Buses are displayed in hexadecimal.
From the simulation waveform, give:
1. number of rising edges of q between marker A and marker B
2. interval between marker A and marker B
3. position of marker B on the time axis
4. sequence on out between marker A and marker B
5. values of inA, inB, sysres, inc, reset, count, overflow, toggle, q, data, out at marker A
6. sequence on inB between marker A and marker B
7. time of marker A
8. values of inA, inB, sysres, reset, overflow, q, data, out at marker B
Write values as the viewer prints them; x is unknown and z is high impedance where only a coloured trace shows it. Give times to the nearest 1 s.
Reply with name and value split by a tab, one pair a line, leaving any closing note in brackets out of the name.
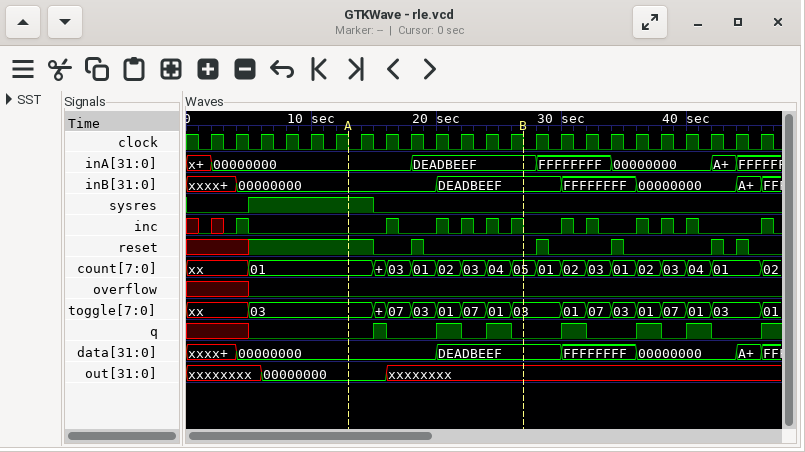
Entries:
number of rising edges of q between marker A and marker B	3
interval between marker A and marker B	14 s
position of marker B on the time axis	27 s
sequence on out between marker A and marker B	00000000, xxxxxxxx
values of inA, inB, sysres, inc, reset, count, overflow, toggle, q, data, out at marker A	inA=00000000, inB=00000000, sysres=1, inc=0, reset=1, count=01, overflow=0, toggle=03, q=0, data=00000000, out=00000000
sequence on inB between marker A and marker B	00000000, DEADBEEF
time of marker A	13 s
values of inA, inB, sysres, reset, overflow, q, data, out at marker B	inA=DEADBEEF, inB=DEADBEEF, sysres=0, reset=0, overflow=0, q=0, data=DEADBEEF, out=xxxxxxxx
